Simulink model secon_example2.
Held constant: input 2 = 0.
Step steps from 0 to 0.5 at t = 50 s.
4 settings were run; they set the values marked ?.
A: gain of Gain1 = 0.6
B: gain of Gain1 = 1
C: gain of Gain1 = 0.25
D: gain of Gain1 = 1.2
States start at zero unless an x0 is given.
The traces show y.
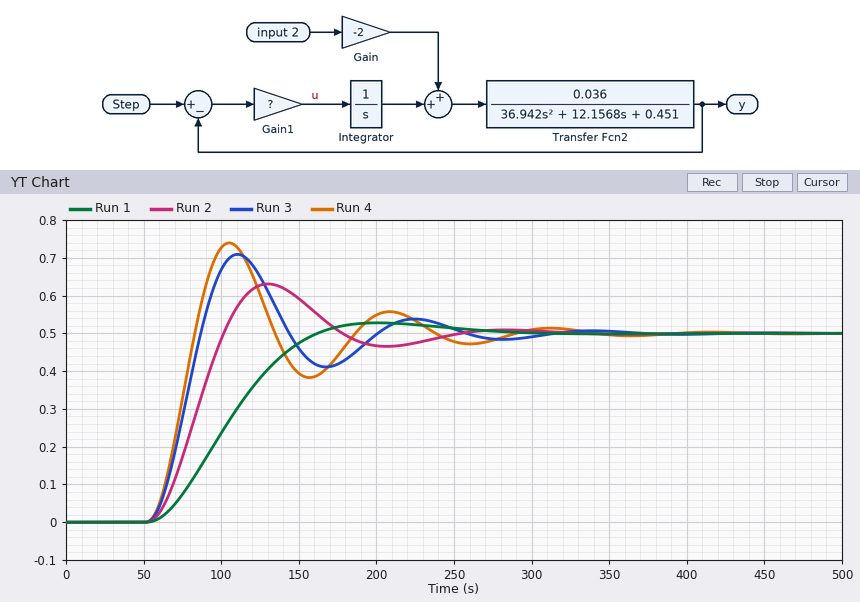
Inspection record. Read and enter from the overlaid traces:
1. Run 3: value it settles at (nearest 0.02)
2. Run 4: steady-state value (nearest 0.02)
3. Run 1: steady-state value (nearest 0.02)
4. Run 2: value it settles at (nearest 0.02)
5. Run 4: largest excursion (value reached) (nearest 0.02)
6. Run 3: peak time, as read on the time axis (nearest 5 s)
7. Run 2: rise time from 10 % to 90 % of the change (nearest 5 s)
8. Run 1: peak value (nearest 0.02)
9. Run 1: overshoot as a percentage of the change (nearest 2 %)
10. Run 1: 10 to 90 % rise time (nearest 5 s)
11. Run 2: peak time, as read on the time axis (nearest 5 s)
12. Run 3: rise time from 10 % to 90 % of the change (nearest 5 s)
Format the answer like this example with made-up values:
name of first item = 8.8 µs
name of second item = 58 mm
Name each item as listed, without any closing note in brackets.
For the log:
Run 3: value it settles at = 0.50
Run 4: steady-state value = 0.50
Run 1: steady-state value = 0.50
Run 2: value it settles at = 0.50
Run 4: largest excursion (value reached) = 0.74
Run 3: peak time, as read on the time axis = 110 s
Run 2: rise time from 10 % to 90 % of the change = 35 s
Run 1: peak value = 0.52
Run 1: overshoot as a percentage of the change = 6 %
Run 1: 10 to 90 % rise time = 70 s
Run 2: peak time, as read on the time axis = 130 s
Run 3: rise time from 10 % to 90 % of the change = 25 s
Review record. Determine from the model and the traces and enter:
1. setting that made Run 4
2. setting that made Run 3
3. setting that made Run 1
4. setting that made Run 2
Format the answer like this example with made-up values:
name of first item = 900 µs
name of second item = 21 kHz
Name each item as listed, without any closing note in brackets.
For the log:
setting that made Run 4 = D
setting that made Run 3 = B
setting that made Run 1 = C
setting that made Run 2 = A
